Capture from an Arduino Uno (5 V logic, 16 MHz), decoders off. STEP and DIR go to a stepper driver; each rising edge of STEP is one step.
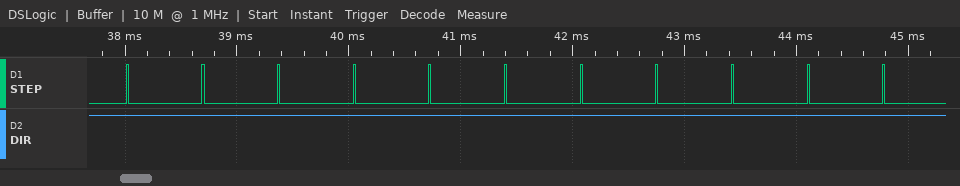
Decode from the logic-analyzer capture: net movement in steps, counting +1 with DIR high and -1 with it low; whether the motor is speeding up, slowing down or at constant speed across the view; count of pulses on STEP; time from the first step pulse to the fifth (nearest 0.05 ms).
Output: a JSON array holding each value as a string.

["+11", "constant speed", "11", "2.70 ms"]
